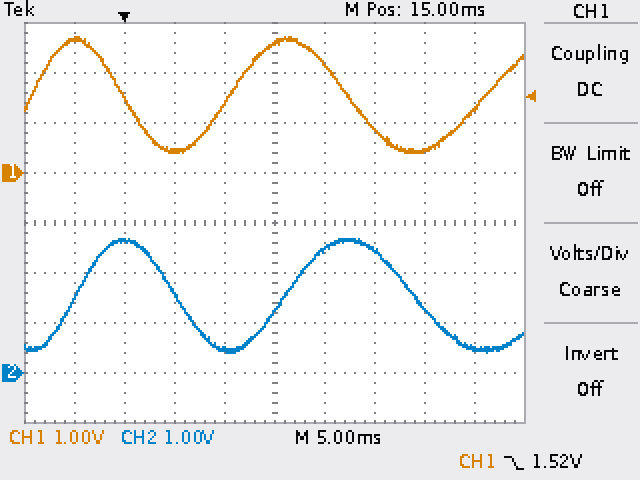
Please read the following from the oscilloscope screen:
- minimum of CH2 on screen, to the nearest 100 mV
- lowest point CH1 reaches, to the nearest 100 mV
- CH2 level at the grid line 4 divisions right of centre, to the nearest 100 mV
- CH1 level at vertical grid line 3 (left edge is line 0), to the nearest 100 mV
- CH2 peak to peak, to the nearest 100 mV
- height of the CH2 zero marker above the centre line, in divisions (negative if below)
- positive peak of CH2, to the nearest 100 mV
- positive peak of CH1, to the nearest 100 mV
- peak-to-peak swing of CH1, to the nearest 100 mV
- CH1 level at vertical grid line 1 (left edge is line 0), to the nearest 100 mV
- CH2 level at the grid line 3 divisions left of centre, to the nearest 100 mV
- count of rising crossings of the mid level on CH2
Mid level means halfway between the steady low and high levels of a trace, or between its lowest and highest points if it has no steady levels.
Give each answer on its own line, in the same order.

400 mV
400 mV
500 mV
400 mV
2.3 V
-3.0 div
2.7 V
2.7 V
2.3 V
2.7 V
2.6 V
2
